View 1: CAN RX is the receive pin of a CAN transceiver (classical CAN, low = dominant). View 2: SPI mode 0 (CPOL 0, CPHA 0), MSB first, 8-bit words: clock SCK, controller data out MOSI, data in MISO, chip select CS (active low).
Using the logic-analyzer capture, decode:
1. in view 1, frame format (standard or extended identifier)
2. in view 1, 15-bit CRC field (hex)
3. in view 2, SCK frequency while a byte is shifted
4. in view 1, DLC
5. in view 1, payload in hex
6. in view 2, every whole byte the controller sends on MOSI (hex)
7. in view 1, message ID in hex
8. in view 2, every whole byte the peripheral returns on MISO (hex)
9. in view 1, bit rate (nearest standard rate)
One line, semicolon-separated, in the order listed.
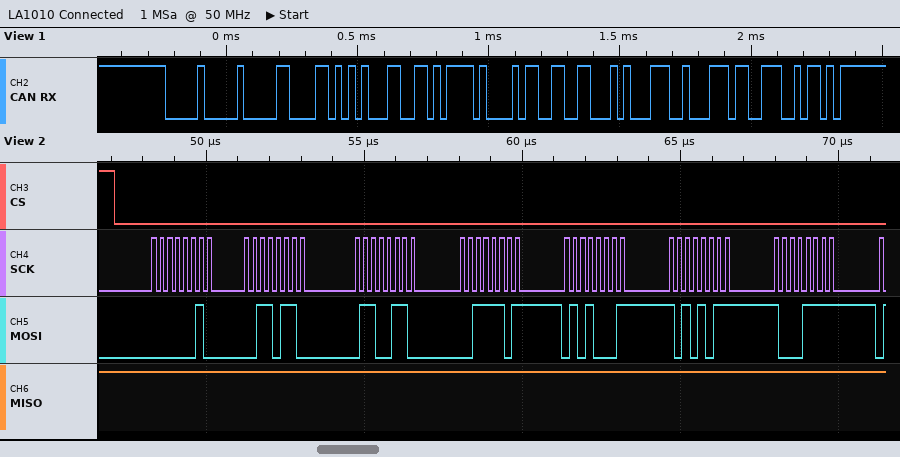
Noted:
standard; 0x3396; 4 MHz; 8; 6A 8C D7 A1 66 62 8E 47; 02 36 66 3D 51 AB 8F; 0x000; FF FF FF FF FF FF FF; 40 kbit/s
